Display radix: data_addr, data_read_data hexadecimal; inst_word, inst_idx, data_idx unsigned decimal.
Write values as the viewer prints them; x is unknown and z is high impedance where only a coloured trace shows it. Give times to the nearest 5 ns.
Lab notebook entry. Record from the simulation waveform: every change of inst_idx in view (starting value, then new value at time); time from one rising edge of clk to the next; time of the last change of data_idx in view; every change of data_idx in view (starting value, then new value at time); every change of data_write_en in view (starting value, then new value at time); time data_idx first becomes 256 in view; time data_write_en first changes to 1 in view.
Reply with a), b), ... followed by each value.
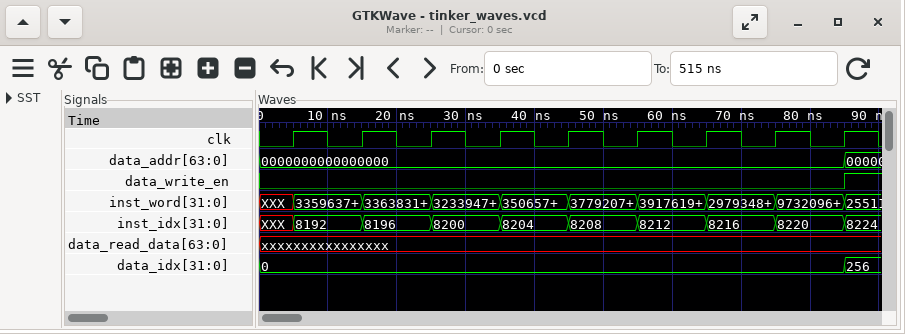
a) XXX, 8192 at 5 ns, 8196 at 15 ns, 8200 at 25 ns, 8204 at 35 ns, 8208 at 45 ns, 8212 at 55 ns, 8216 at 65 ns, 8220 at 75 ns, 8224 at 85 ns
b) 10 ns
c) 85 ns
d) 0, 256 at 85 ns
e) 0, 1 at 85 ns
f) 85 ns
g) 85 ns
